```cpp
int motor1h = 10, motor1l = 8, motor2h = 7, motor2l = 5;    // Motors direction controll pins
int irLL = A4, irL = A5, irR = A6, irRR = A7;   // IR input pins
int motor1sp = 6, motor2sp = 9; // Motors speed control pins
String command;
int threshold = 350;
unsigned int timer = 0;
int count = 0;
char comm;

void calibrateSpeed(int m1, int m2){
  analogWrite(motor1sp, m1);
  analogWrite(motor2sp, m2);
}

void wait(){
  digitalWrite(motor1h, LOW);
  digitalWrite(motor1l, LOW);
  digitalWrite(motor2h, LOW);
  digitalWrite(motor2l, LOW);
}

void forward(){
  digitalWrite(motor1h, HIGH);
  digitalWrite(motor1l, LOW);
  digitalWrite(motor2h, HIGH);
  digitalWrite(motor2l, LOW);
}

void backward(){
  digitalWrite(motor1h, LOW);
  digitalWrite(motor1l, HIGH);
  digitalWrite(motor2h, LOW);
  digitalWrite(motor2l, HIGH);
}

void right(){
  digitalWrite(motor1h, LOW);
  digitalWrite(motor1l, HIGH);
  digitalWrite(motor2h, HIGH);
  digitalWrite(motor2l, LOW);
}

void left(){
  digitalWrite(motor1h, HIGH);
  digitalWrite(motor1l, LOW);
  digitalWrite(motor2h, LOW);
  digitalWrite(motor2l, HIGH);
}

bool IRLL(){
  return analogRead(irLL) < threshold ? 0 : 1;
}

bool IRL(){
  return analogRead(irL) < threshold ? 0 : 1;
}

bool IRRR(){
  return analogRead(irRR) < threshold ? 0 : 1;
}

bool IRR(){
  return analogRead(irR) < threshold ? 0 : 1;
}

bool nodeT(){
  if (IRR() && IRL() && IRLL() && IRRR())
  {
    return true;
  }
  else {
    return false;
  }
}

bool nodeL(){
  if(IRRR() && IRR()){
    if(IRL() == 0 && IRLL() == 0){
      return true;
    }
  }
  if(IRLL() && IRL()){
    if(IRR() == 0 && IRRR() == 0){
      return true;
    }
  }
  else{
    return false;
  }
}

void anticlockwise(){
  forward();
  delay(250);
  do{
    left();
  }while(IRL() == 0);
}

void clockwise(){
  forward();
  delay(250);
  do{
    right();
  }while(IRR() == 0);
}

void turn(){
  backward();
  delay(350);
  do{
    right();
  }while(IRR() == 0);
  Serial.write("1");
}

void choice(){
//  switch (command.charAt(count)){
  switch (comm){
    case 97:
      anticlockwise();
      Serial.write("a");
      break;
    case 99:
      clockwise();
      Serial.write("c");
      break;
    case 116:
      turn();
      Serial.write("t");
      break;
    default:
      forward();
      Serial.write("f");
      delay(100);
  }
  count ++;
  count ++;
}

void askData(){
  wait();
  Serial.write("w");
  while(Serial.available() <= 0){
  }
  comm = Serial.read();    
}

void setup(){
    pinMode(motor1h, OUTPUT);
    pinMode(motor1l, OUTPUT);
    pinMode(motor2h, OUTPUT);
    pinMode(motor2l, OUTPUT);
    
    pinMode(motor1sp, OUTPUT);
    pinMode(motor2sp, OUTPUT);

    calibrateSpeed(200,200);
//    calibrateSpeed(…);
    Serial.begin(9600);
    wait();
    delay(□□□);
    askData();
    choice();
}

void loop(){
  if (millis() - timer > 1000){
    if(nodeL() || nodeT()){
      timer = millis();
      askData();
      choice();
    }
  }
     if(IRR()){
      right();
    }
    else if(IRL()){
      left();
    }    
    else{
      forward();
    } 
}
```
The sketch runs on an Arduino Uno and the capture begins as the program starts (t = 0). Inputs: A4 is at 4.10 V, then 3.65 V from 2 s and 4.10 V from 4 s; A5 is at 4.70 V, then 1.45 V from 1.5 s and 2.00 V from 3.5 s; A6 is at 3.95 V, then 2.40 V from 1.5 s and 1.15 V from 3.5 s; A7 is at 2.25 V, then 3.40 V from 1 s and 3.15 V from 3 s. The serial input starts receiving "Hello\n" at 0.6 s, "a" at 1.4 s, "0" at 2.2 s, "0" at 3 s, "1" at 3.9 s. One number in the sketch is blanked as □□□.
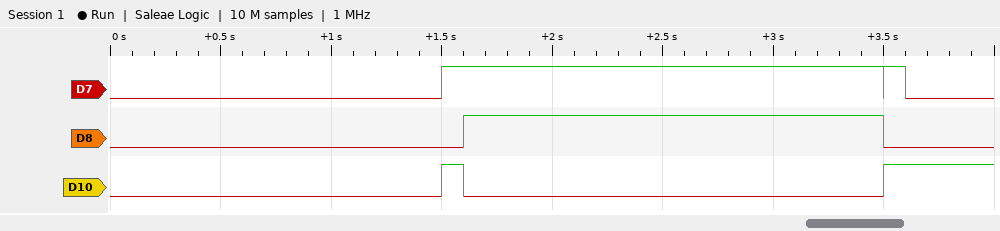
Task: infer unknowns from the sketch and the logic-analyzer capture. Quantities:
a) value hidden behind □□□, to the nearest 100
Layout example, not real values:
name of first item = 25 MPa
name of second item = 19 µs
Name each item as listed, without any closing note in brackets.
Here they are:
value hidden behind □□□, to the nearest 100 = 1500
